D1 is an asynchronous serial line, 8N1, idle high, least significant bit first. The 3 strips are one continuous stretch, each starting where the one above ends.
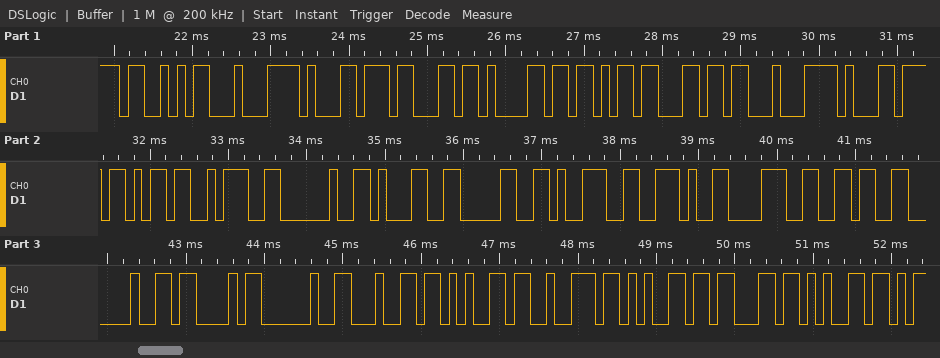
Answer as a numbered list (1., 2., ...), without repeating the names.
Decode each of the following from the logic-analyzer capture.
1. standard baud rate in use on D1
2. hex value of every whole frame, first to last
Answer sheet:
1. 9600 baud
2. 53 C4 B1 63 61 6B 6C C4 B1 6B 3A 20 31 30 39 2E 38 36 20 43 20 64 65 72 65 63 65
